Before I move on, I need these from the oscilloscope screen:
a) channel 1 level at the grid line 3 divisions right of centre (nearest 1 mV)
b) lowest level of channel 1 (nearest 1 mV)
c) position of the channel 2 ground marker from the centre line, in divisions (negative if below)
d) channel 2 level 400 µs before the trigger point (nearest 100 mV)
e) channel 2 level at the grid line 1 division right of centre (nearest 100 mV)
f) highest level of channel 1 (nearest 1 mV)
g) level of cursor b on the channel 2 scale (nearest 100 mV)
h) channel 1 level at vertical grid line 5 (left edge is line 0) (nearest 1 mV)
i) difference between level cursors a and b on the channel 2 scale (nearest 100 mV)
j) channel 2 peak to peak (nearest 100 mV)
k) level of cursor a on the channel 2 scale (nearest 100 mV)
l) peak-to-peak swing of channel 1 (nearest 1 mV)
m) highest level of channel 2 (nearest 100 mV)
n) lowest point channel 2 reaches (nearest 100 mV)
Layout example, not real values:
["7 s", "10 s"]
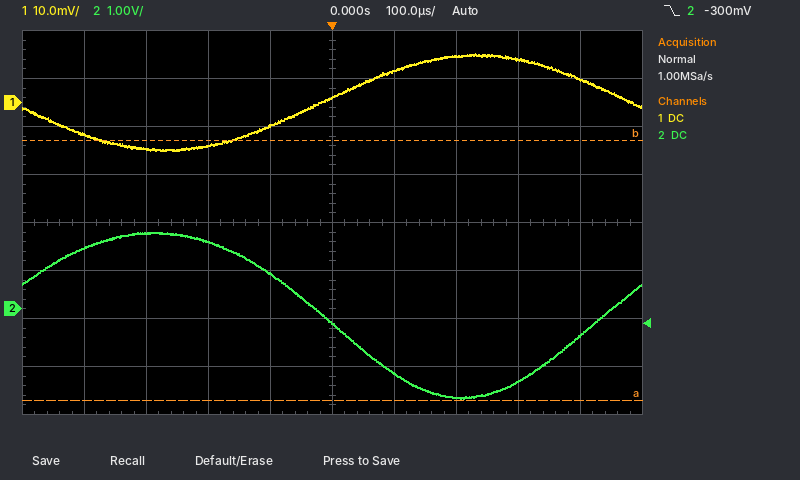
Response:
["9 mV", "-10 mV", "-1.8 div", "1.3 V", "-1.3 V", "10 mV", "3.5 V", "1 mV", "5.4 V", "3.5 V", "-1.9 V", "20 mV", "1.6 V", "-1.9 V"]
